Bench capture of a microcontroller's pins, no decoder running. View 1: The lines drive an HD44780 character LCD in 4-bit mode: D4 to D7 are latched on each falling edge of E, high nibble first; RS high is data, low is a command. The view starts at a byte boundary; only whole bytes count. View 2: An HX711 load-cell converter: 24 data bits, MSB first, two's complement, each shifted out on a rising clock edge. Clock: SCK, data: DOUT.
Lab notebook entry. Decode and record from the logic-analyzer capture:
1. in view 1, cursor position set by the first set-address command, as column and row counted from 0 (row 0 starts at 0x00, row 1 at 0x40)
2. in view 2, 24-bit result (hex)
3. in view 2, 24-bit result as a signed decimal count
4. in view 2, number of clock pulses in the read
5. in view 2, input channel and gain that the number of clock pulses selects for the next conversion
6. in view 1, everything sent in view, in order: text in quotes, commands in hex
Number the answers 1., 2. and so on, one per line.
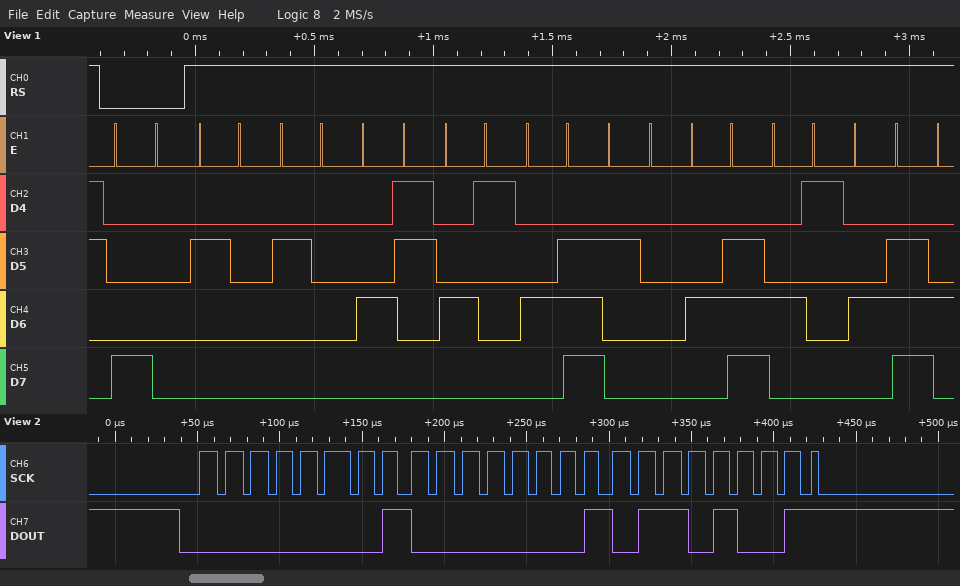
1. column 0, row 0
2. 0x010169
3. 65897
4. 25
5. channel A, gain 128
6. 0x80 "  CAN NAN"
